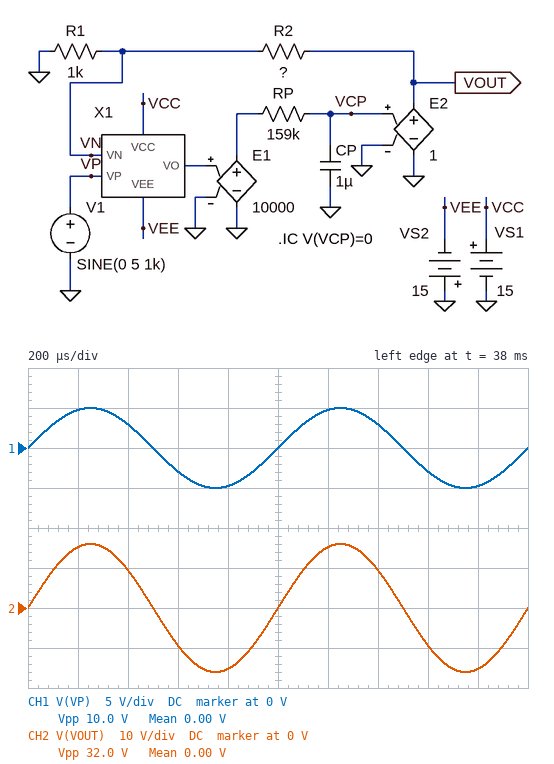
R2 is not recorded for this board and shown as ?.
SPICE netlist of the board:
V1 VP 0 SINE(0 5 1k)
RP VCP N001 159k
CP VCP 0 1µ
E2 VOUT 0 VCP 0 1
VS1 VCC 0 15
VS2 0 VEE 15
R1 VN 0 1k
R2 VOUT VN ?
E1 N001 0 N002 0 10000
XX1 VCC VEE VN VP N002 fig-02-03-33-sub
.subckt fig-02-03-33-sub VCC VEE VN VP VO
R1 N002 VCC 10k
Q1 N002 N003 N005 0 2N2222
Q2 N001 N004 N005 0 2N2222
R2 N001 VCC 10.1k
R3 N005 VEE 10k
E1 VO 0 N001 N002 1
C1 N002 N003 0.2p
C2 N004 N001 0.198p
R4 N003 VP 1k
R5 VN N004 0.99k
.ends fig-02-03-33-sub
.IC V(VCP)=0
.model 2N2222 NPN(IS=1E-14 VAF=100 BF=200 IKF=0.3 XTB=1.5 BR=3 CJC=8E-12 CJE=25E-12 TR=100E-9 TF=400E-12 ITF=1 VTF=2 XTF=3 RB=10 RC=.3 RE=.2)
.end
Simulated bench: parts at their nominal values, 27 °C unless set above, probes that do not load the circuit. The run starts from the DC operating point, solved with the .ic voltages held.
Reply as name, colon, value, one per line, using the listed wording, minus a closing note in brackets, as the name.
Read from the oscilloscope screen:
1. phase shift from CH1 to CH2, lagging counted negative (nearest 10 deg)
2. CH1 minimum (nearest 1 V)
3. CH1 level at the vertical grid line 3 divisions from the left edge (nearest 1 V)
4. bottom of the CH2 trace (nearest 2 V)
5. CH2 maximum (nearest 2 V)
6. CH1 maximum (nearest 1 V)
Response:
phase shift from CH1 to CH2, lagging counted negative: 0 deg
CH1 minimum: -5 V
CH1 level at the vertical grid line 3 divisions from the left edge: -3 V
bottom of the CH2 trace: -16 V
CH2 maximum: 16 V
CH1 maximum: 5 V
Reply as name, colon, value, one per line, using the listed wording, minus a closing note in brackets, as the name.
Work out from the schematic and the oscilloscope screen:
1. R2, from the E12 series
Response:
R2, from the E12 series: 2.2 kΩ
